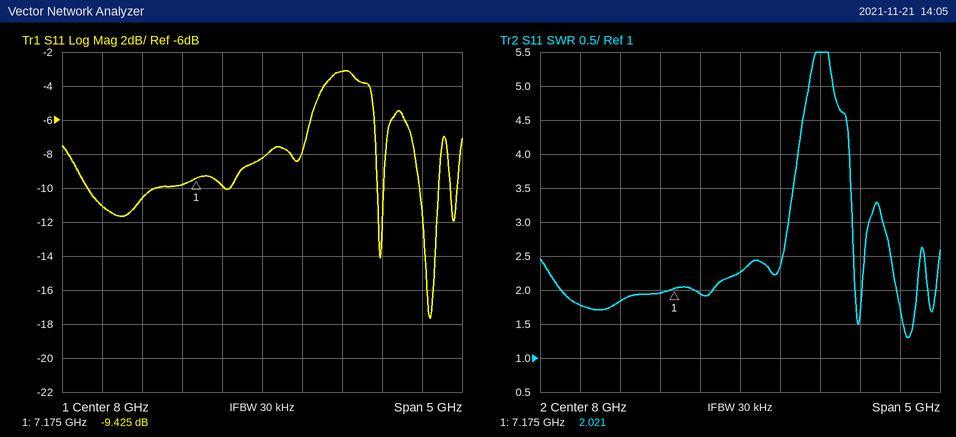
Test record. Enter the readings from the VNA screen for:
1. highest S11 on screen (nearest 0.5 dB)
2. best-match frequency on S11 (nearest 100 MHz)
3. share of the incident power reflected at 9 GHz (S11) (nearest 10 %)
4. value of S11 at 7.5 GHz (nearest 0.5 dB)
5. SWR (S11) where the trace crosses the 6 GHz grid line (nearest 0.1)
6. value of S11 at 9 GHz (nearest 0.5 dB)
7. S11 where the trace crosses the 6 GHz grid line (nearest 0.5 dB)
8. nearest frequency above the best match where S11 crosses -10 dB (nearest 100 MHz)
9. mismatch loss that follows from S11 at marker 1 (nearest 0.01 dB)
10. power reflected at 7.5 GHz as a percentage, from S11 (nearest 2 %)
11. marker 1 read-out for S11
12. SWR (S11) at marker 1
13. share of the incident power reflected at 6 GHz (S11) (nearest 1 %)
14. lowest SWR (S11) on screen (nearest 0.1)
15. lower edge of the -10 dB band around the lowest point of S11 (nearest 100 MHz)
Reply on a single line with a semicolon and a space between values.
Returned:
-3.0 dB; 10.1 GHz; 50 %; -10.0 dB; 1.8; -3.0 dB; -11.0 dB; 10.2 GHz; 0.53 dB; 10 %; -9.425 dB; 2.021; 8 %; 1.3; 10.0 GHz
